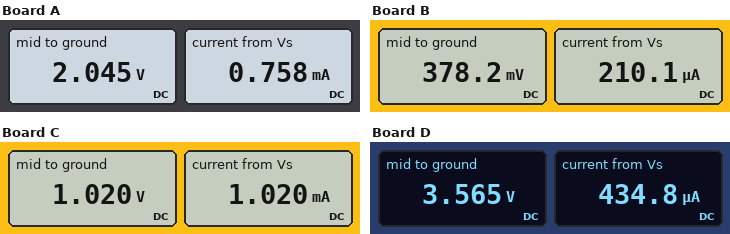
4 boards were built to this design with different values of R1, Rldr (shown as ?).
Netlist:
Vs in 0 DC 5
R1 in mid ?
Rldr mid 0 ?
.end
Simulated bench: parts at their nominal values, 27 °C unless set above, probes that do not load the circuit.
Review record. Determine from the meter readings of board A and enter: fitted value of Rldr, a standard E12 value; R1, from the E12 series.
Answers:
2.7 kΩ
3.9 kΩ
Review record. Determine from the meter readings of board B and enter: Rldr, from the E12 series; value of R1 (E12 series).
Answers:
1.8 kΩ
22 kΩ
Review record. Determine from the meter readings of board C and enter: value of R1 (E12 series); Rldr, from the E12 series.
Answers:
3.9 kΩ
1 kΩ
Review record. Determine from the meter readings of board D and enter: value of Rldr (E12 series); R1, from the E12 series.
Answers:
8.2 kΩ
3.3 kΩ
